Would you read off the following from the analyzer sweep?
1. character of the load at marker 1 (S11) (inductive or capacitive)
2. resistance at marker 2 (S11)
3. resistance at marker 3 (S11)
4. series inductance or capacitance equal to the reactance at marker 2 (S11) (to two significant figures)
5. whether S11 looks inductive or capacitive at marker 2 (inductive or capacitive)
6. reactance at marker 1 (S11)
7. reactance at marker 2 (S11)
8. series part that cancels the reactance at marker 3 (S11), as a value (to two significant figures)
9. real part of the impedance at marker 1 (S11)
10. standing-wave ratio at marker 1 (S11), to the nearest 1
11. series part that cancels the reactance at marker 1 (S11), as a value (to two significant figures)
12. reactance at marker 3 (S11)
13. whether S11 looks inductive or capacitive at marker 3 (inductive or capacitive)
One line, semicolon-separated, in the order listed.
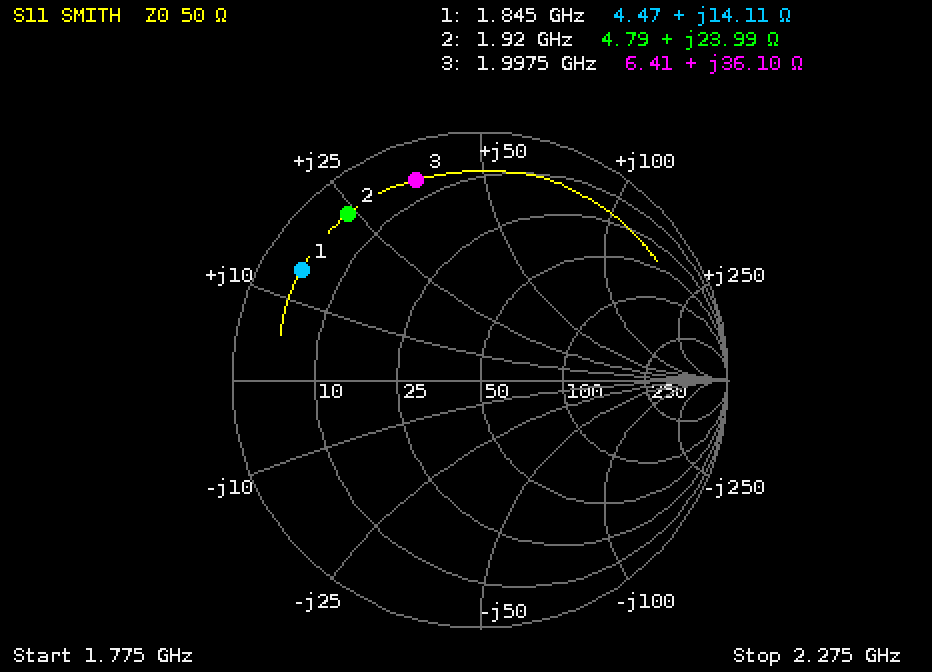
inductive; 4.79 Ω; 6.41 Ω; 2.0 nH; inductive; +14.11 Ω; +23.99 Ω; 2.2 pF; 4.47 Ω; 12; 6.1 pF; +36.10 Ω; inductive
